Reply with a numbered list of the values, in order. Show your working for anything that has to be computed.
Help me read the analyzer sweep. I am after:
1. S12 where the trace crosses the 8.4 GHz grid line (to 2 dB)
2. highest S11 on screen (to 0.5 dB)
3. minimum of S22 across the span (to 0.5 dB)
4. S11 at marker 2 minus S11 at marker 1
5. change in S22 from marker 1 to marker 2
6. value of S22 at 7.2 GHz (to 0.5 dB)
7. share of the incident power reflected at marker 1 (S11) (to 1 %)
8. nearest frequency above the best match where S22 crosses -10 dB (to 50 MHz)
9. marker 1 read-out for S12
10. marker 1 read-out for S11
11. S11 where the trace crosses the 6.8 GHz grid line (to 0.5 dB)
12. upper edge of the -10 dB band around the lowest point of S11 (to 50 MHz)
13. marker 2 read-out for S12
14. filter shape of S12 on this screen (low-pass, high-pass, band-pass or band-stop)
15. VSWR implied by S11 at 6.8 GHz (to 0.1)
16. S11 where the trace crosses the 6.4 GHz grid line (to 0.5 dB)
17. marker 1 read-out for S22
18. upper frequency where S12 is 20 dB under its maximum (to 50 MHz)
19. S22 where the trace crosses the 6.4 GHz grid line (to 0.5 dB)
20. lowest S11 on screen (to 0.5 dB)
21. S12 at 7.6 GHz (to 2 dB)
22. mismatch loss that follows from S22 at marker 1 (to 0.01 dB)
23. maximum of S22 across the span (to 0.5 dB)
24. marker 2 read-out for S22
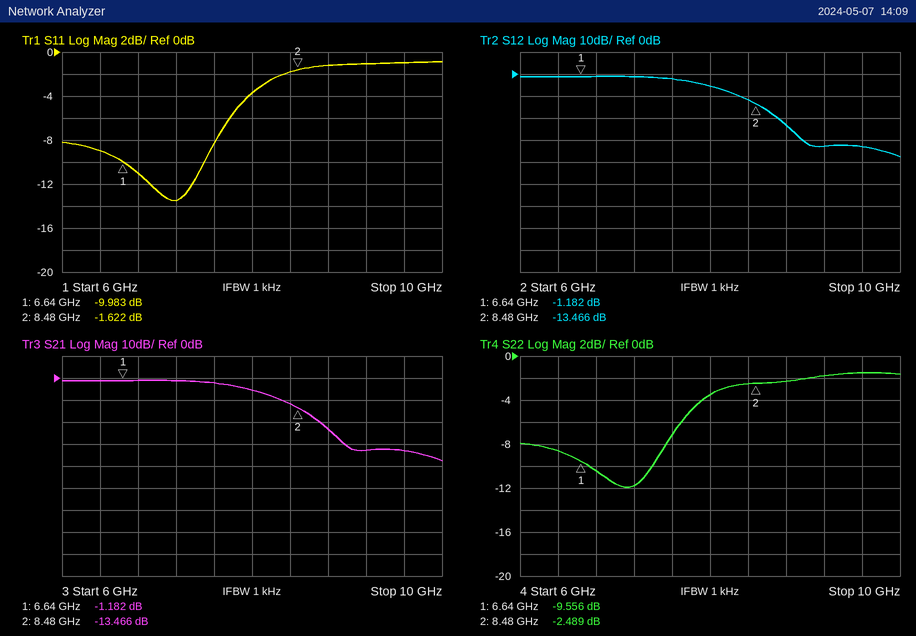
1. -12 dB
2. -1.0 dB
3. -12.0 dB
4. -1.622 − (-9.983) = 8.361 dB
5. -2.489 − (-9.556) = 7.067 dB
6. -12.0 dB
7. 10^(-9.983/10) ≈ 10 %
8. 7.40 GHz
9. -1.182 dB
10. -9.983 dB
11. -11.0 dB
12. 7.50 GHz
13. -13.466 dB
14. low-pass
15. |Γ| = 10^(-11/20) = 0.2818; VSWR = (1 + 0.2818)/(1 − 0.2818) ≈ 1.8
16. -9.0 dB
17. -9.556 dB
18. 8.75 GHz
19. -8.5 dB
20. -13.5 dB
21. -2 dB
22. −10 log10(1 − 10^(-9.556/10)) ≈ 0.51 dB
23. -1.5 dB
24. -2.489 dB
